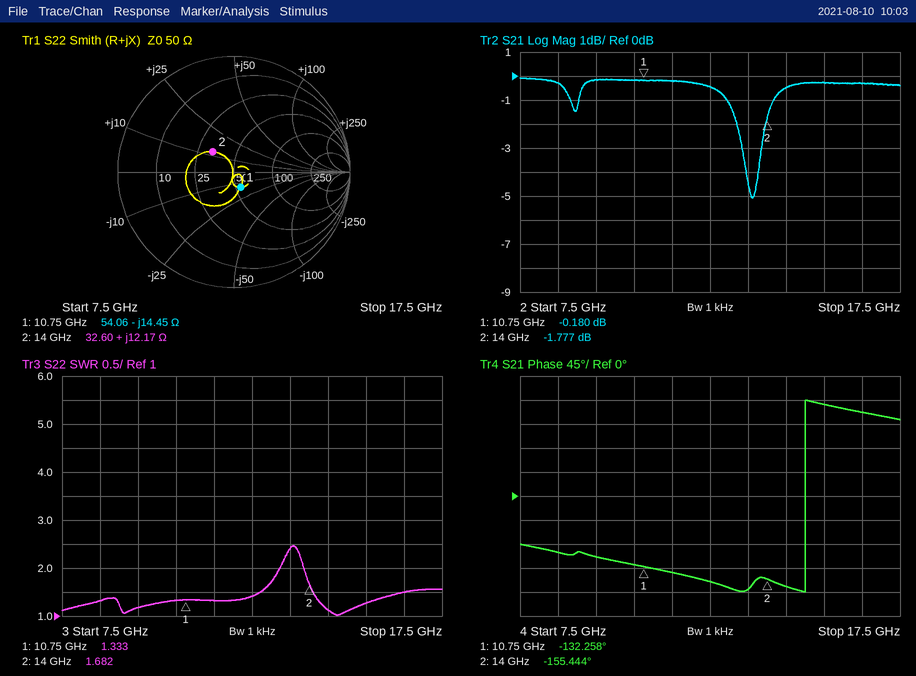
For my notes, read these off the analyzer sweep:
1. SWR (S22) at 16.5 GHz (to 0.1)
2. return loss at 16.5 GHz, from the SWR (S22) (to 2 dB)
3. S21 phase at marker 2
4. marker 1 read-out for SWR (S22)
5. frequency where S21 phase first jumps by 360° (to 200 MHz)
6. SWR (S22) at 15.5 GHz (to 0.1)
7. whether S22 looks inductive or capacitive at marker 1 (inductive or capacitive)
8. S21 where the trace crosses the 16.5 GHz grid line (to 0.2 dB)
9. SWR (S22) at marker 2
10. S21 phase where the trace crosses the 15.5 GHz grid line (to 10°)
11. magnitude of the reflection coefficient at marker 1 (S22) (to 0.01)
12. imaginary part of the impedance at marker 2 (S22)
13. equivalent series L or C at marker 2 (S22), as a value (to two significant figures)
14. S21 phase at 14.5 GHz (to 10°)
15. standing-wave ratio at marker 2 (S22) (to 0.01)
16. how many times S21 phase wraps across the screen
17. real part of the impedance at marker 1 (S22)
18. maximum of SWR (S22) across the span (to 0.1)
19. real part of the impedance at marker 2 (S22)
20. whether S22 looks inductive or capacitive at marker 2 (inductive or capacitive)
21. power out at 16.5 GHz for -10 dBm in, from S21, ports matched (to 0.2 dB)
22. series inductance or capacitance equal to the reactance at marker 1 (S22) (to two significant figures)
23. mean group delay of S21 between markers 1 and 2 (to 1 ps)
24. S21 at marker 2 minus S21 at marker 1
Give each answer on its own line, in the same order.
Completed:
1.5
14 dB
-155.444°
1.333
15.0 GHz
1.3
capacitive
-0.4 dB
1.682
170°
0.14
+12.17 Ω
140 pH
-170°
1.68
1
54.06 Ω
2.5
32.60 Ω
inductive
-10.4 dBm
1.0 pF
20 ps
-1.597 dB
